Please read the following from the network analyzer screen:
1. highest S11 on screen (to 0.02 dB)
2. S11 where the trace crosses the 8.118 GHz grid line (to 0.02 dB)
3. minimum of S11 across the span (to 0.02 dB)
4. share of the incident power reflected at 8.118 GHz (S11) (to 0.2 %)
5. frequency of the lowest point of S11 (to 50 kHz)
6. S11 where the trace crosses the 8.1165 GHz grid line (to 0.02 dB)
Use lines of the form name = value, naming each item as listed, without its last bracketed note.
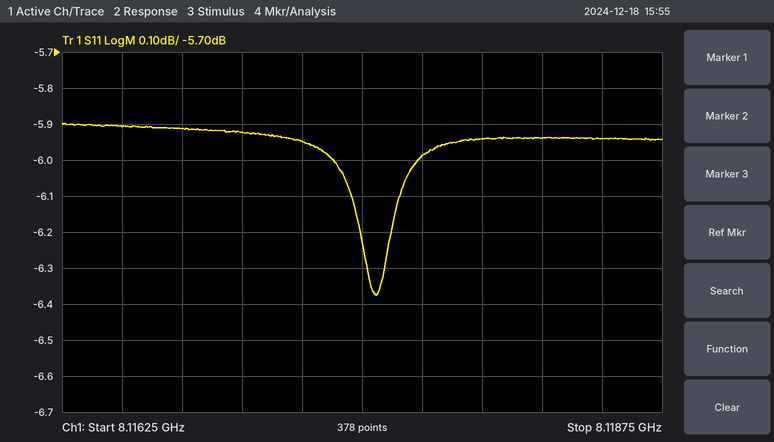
highest S11 on screen = -5.90 dB
S11 where the trace crosses the 8.118 GHz grid line = -5.94 dB
minimum of S11 across the span = -6.38 dB
share of the incident power reflected at 8.118 GHz (S11) = 25.4 %
frequency of the lowest point of S11 = 8.11755 GHz
S11 where the trace crosses the 8.1165 GHz grid line = -5.90 dB
